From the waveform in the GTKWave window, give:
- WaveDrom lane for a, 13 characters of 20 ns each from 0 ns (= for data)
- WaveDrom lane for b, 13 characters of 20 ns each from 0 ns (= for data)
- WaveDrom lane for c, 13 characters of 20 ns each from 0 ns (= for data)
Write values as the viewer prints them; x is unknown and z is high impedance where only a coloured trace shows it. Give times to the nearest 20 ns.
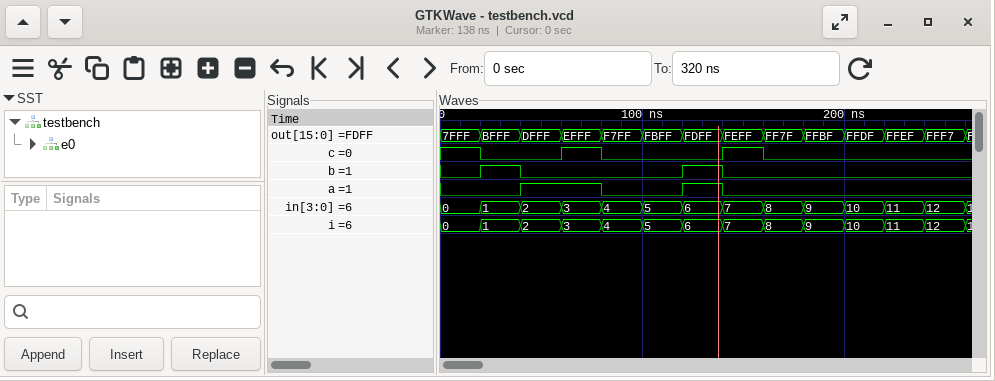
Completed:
{name: 'a', wave: '0.1.0.10.....'}
{name: 'b', wave: '010...10.....'}
{name: 'c', wave: '10.10..10....'}
